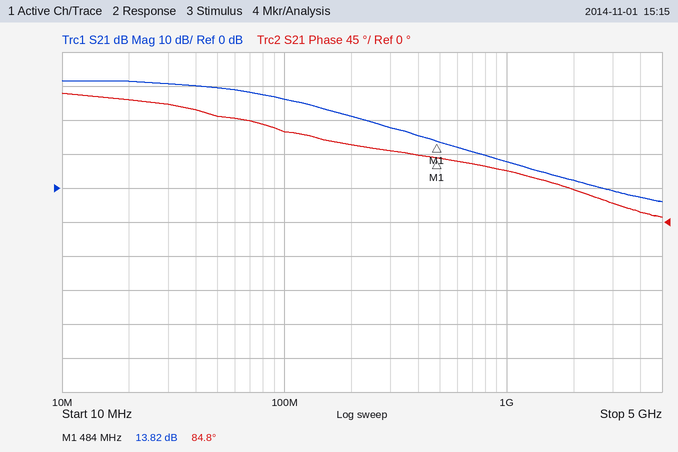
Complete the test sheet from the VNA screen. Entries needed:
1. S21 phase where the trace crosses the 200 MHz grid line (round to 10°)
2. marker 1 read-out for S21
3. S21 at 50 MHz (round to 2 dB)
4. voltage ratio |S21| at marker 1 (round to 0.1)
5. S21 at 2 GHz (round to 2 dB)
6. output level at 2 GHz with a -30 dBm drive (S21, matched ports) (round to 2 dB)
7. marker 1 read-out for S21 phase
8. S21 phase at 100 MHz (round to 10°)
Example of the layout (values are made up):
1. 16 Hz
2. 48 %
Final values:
1. 100°
2. 13.82 dB
3. 30 dB
4. 4.9
5. 2 dB
6. -28 dBm
7. 84.8°
8. 120°
